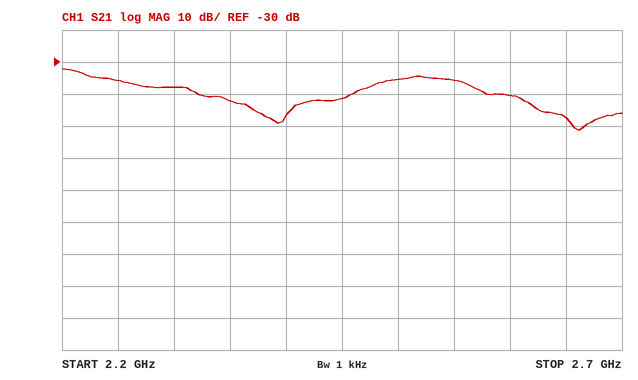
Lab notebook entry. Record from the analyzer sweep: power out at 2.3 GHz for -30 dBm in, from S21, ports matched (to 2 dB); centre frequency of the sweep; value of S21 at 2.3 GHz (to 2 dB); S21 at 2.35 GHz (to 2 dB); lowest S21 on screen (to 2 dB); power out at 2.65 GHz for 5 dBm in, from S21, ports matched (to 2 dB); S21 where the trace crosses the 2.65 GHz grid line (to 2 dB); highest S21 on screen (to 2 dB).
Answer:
-68 dBm
2.45 GHz
-38 dB
-42 dB
-52 dB
-42 dBm
-48 dB
-32 dB
